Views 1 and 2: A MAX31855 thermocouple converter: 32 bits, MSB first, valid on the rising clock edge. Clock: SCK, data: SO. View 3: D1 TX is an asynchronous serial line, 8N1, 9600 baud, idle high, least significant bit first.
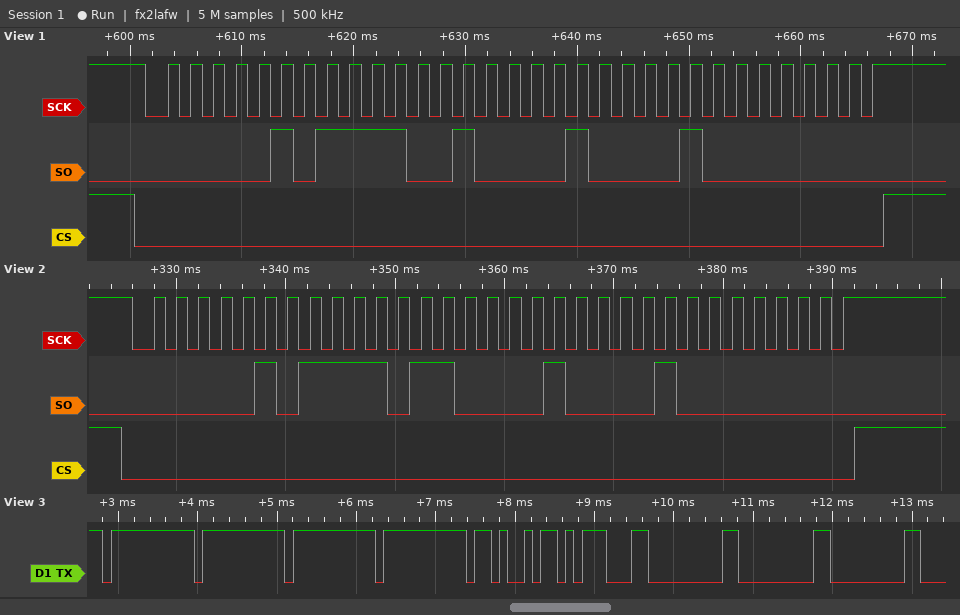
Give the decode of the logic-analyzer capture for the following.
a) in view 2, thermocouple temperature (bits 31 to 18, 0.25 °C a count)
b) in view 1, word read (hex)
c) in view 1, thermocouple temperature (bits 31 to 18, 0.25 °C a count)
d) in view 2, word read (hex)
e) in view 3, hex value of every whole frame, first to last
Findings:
94.75 °C
0x05E42100
94.25 °C
0x05EC2100
0xFF 0xFF 0xFF 0xFF 0x4B 0x1D 0x00 0x00 0x00
